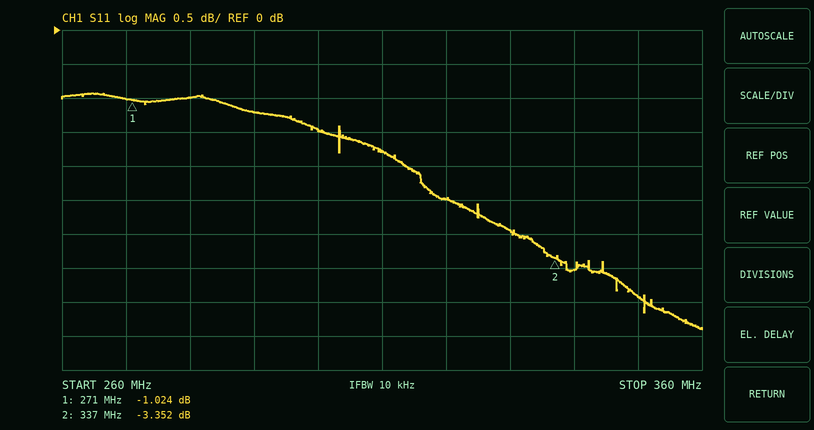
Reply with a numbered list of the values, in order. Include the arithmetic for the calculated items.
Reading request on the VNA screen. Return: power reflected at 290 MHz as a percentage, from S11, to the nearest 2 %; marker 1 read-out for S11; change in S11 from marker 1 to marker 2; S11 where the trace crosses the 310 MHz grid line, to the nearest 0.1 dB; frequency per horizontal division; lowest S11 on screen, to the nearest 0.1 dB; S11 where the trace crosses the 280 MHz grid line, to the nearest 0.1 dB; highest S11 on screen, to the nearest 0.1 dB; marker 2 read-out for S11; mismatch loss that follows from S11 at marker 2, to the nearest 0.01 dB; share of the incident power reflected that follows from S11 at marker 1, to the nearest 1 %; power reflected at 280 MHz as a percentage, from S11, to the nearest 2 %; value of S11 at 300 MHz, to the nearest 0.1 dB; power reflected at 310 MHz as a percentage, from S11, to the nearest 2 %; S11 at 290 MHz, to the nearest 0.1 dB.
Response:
1. 10^(-1.2/10) ≈ 76 %
2. -1.024 dB
3. -3.352 − (-1.024) = -2.328 dB
4. -1.8 dB
5. 10 MHz
6. -4.4 dB
7. -1.0 dB
8. -0.9 dB
9. -3.352 dB
10. −10 log10(1 − 10^(-3.352/10)) ≈ 2.69 dB
11. 10^(-1.024/10) ≈ 79 %
12. 10^(-1/10) ≈ 79.4 %, so 80 % to the nearest 2 %
13. -1.5 dB
14. 10^(-1.8/10) ≈ 66 %
15. -1.2 dB
